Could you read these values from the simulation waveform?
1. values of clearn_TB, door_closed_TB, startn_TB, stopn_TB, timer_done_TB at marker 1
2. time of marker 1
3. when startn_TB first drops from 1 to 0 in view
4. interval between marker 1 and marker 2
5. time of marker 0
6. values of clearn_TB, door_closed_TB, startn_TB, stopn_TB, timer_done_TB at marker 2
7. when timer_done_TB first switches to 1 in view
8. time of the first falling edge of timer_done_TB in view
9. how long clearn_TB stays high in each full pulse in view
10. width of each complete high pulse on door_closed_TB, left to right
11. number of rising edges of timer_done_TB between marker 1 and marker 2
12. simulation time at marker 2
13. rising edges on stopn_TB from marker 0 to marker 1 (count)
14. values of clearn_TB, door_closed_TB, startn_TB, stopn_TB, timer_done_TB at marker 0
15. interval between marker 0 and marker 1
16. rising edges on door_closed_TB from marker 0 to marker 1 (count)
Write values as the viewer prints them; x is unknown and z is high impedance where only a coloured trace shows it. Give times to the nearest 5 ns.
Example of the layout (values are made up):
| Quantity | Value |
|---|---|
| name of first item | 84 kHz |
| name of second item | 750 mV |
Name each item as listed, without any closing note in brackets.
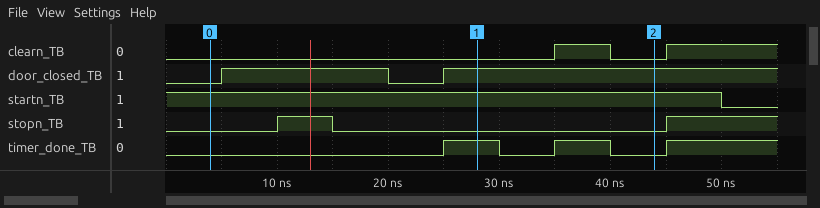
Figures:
| Quantity | Value |
|---|---|
| values of clearn_TB, door_closed_TB, startn_TB, stopn_TB, timer_done_TB at marker 1 | clearn_TB=0, door_closed_TB=1, startn_TB=1, stopn_TB=0, timer_done_TB=1 |
| time of marker 1 | 30 ns |
| when startn_TB first drops from 1 to 0 in view | 50 ns |
| interval between marker 1 and marker 2 | 15 ns |
| time of marker 0 | 5 ns |
| values of clearn_TB, door_closed_TB, startn_TB, stopn_TB, timer_done_TB at marker 2 | clearn_TB=0, door_closed_TB=1, startn_TB=1, stopn_TB=0, timer_done_TB=0 |
| when timer_done_TB first switches to 1 in view | 25 ns |
| time of the first falling edge of timer_done_TB in view | 30 ns |
| how long clearn_TB stays high in each full pulse in view | 5 ns |
| width of each complete high pulse on door_closed_TB, left to right | 15 ns |
| number of rising edges of timer_done_TB between marker 1 and marker 2 | 1 |
| simulation time at marker 2 | 45 ns |
| rising edges on stopn_TB from marker 0 to marker 1 | 1 |
| values of clearn_TB, door_closed_TB, startn_TB, stopn_TB, timer_done_TB at marker 0 | clearn_TB=0, door_closed_TB=0, startn_TB=1, stopn_TB=0, timer_done_TB=0 |
| interval between marker 0 and marker 1 | 25 ns |
| rising edges on door_closed_TB from marker 0 to marker 1 | 2 |
